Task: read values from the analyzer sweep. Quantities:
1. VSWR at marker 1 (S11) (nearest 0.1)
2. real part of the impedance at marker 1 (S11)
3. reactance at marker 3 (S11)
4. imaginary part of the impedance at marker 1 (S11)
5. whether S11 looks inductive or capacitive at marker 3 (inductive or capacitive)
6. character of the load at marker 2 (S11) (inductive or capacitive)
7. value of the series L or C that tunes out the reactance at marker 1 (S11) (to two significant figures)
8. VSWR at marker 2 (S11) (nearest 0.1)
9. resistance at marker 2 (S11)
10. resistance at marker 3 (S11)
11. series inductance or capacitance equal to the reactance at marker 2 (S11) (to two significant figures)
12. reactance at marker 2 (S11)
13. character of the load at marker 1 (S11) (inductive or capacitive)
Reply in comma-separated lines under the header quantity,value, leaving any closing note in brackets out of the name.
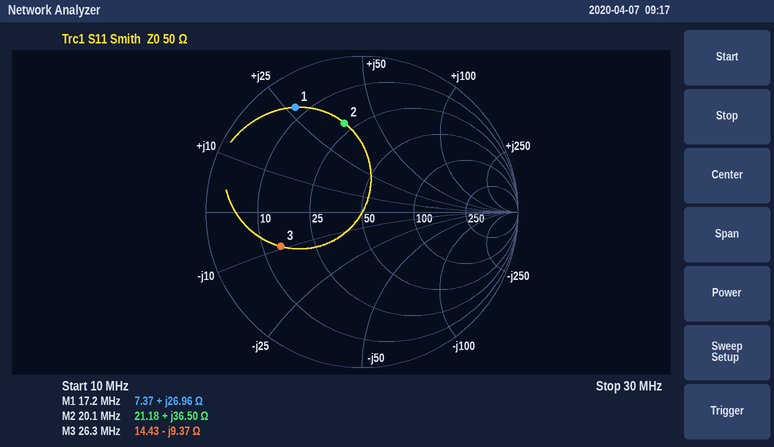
quantity,value
VSWR at marker 1 (S11),8.8
real part of the impedance at marker 1,7.37 Ω
reactance at marker 3,-9.37 Ω
imaginary part of the impedance at marker 1,+26.96 Ω
whether S11 looks inductive or capacitive at marker 3,capacitive
character of the load at marker 2 (S11),inductive
value of the series L or C that tunes out the reactance at marker 1 (S11),340 pF
VSWR at marker 2 (S11),3.8
resistance at marker 2,21.18 Ω
resistance at marker 3,14.43 Ω
series inductance or capacitance equal to the reactance at marker 2 (S11),290 nH
reactance at marker 2,+36.50 Ω
character of the load at marker 1 (S11),inductive
